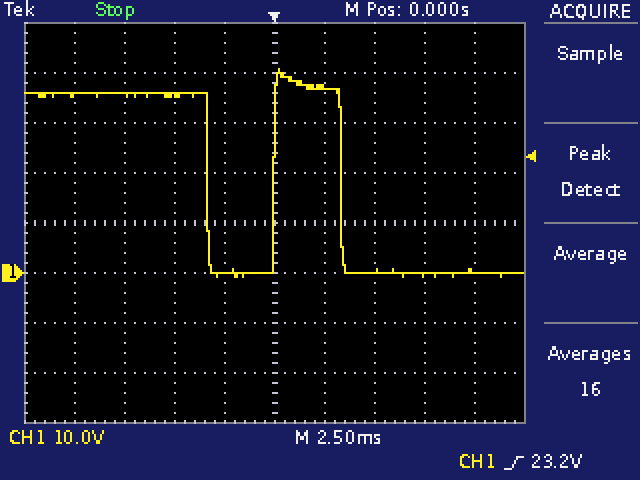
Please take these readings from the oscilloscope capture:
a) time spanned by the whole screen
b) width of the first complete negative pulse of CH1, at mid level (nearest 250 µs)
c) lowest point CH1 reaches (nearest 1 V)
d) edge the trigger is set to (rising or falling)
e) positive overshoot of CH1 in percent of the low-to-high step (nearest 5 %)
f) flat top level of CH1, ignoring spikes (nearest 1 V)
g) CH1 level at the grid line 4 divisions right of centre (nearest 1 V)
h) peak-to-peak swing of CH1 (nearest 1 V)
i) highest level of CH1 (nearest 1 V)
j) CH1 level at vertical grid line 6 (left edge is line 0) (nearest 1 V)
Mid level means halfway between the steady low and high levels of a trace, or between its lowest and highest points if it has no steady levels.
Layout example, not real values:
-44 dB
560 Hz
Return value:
25 ms
3.25 ms
-1 V
rising
15 %
36 V
0 V
42 V
41 V
37 V
